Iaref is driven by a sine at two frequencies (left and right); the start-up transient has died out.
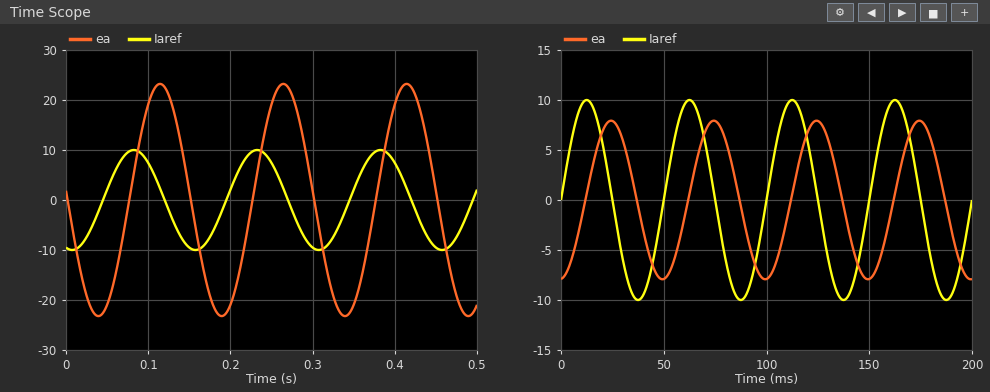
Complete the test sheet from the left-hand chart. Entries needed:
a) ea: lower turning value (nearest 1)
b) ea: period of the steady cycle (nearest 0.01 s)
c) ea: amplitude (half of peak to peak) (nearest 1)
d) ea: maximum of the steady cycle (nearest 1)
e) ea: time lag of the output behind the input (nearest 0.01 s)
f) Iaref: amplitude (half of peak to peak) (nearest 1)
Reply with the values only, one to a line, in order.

-23
0.15 s
23
23
0.03 s
10
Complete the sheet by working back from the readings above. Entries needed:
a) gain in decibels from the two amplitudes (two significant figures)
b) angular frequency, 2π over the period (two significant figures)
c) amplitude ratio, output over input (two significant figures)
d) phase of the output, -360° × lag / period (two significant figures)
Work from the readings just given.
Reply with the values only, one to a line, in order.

7.2 dB
42 rad/s
2.3
-72°
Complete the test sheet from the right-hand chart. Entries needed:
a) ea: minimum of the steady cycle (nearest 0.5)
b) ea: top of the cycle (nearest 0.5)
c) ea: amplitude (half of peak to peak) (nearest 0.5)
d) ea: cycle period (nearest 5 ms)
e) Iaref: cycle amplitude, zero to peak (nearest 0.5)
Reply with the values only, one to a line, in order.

-8.0
8.0
8.0
50 ms
10.0
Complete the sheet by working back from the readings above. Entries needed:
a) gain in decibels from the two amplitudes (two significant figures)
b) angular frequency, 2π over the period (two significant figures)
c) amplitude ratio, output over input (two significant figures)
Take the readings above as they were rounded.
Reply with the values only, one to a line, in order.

-1.9 dB
0.13 rad/ms
0.80
